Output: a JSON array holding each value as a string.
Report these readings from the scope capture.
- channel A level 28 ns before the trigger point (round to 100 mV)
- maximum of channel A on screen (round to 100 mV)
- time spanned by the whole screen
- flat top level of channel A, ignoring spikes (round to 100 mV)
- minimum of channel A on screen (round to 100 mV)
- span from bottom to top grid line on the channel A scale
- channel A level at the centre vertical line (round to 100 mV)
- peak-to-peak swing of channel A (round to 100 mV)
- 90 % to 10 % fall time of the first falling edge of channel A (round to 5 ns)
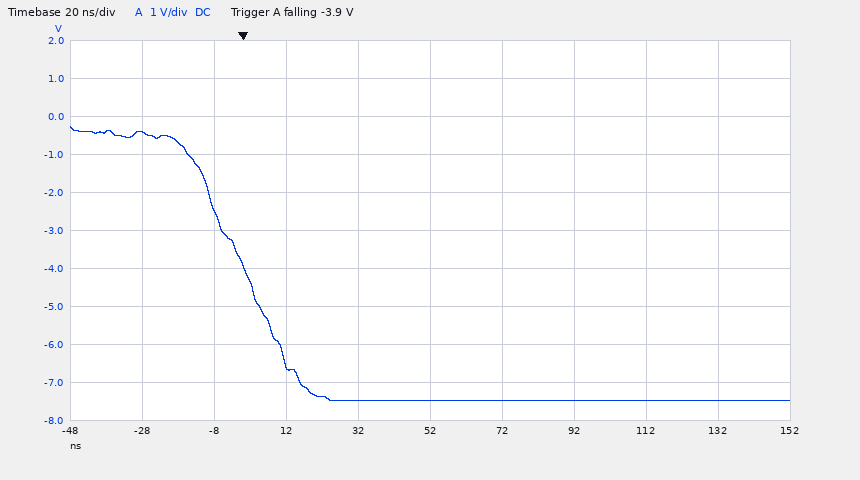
["-400 mV", "-300 mV", "200 ns", "-400 mV", "-7.5 V", "10 V", "-7.5 V", "7.2 V", "30 ns"]
